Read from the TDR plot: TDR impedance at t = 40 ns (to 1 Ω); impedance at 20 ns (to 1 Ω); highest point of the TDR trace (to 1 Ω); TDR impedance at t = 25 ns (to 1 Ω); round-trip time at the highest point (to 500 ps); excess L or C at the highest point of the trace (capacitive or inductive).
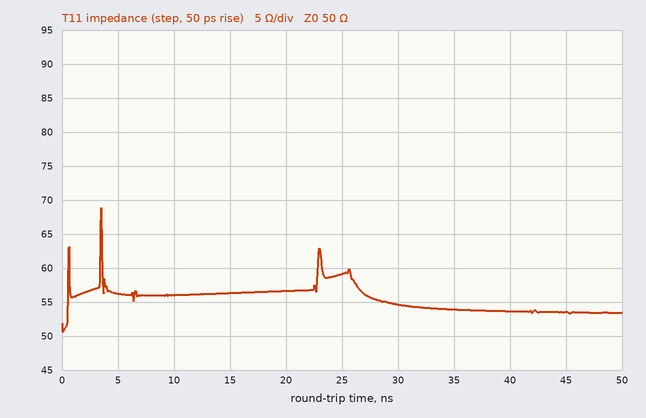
54 Ω
57 Ω
69 Ω
59 Ω
3.5 ns
inductive
